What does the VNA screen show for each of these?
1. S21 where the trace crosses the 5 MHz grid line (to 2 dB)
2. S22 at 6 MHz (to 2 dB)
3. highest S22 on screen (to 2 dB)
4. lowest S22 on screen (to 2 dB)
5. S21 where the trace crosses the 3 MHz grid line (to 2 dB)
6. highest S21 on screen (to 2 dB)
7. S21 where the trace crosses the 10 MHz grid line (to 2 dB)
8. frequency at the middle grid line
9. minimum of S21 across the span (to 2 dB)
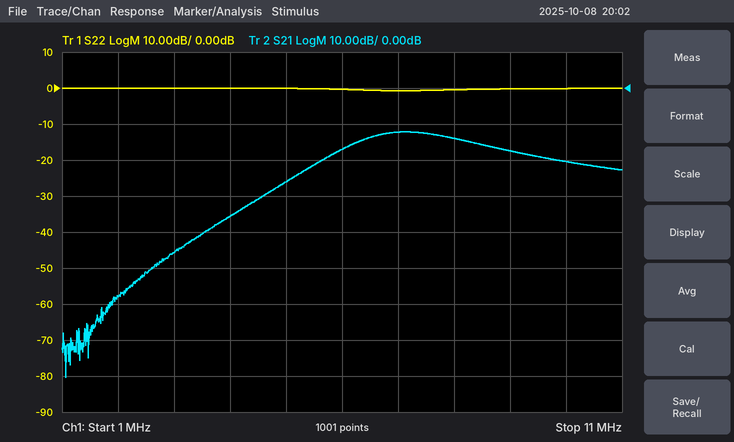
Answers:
-26 dB
0 dB
0 dB
0 dB
-46 dB
-12 dB
-20 dB
6 MHz
-80 dB
